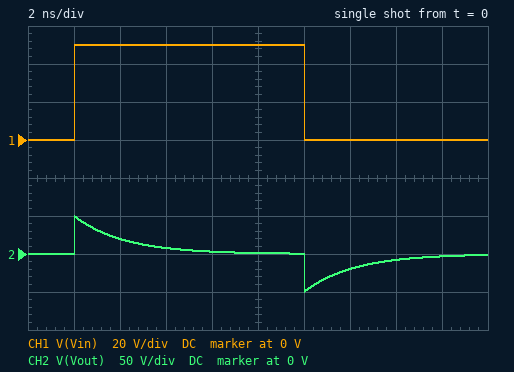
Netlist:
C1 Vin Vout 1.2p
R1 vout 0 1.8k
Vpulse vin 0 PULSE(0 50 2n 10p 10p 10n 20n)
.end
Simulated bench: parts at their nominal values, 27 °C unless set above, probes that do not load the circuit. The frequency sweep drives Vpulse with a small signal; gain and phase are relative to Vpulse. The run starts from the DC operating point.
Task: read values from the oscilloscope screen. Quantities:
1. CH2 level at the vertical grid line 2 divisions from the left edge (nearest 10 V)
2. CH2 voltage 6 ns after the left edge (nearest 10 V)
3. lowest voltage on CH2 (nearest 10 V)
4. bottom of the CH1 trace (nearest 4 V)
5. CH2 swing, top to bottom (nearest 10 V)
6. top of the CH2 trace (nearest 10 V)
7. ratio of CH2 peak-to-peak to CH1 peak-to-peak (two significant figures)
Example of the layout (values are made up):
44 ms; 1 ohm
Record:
20 V; 10 V; -50 V; 0 V; 100 V; 50 V; 2.0
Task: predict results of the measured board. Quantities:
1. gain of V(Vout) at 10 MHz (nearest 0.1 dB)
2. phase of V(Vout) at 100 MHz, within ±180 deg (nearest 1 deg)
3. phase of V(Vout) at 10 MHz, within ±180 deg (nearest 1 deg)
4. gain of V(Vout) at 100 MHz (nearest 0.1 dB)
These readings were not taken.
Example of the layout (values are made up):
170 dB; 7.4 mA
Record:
-17.4 dB; 36 deg; 82 deg; -1.9 dB
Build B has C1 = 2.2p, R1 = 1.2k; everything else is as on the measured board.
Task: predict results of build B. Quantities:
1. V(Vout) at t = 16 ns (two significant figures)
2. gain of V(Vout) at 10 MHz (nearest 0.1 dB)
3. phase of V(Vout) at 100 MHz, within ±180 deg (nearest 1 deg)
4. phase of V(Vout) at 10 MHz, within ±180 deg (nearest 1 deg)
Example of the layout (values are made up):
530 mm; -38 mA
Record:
-11 V; -15.7 dB; 31 deg; 81 deg
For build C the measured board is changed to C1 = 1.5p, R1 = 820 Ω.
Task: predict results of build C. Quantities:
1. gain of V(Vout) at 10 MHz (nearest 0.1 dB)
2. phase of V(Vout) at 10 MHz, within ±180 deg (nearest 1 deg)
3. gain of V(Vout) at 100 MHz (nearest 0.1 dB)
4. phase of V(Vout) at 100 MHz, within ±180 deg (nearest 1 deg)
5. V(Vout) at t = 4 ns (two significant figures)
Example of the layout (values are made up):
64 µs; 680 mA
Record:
-22.3 dB; 86 deg; -4.3 dB; 52 deg; 9.9 V
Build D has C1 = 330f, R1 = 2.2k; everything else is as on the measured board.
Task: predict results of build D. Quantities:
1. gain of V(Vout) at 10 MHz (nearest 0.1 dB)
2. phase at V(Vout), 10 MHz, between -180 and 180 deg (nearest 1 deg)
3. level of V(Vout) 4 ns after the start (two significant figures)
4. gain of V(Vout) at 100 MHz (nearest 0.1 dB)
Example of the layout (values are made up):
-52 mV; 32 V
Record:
-26.8 dB; 87 deg; 3.2 V; -7.6 dB
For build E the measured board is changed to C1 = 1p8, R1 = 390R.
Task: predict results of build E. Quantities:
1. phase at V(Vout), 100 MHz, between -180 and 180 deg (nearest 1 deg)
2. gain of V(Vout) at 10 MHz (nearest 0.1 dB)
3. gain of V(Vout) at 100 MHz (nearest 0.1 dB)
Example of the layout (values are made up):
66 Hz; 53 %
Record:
66 deg; -27.1 dB; -7.9 dB
